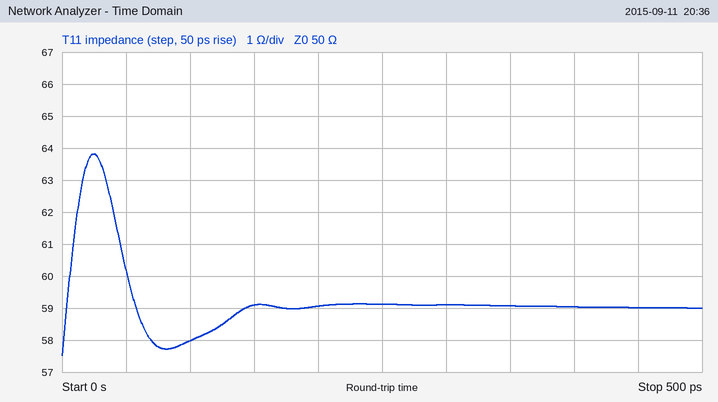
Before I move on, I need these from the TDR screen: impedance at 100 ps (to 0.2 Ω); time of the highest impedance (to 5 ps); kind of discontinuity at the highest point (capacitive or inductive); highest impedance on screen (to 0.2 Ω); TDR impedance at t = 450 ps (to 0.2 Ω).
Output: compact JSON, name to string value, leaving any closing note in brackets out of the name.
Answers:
{"impedance at 100 ps": "58.0 Ω", "time of the highest impedance": "25 ps", "kind of discontinuity at the highest point": "inductive", "highest impedance on screen": "63.8 Ω", "TDR impedance at t = 450 ps": "59.0 Ω"}
